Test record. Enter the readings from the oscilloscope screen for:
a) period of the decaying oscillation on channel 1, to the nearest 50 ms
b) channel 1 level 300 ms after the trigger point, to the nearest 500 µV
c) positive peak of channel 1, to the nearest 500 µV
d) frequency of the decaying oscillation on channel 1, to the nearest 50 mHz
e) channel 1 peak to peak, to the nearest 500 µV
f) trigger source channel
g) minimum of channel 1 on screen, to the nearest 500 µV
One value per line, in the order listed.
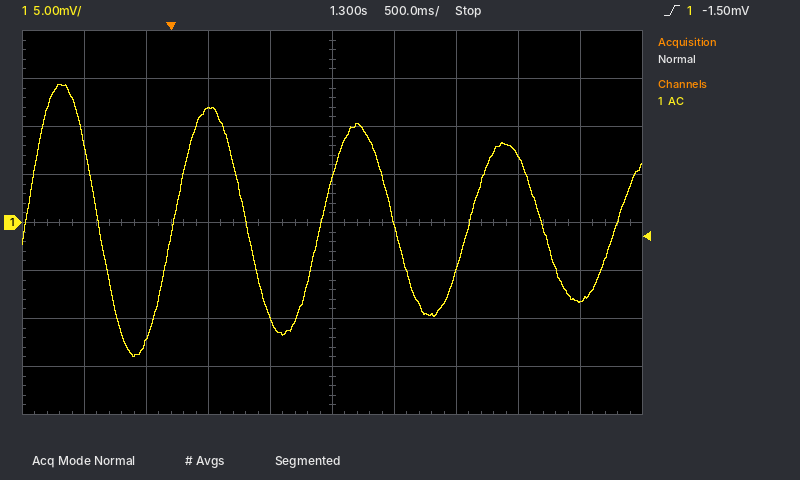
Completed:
1.20 s
12.0 mV
14.5 mV
850 mHz
28.5 mV
channel 1
-14.0 mV
